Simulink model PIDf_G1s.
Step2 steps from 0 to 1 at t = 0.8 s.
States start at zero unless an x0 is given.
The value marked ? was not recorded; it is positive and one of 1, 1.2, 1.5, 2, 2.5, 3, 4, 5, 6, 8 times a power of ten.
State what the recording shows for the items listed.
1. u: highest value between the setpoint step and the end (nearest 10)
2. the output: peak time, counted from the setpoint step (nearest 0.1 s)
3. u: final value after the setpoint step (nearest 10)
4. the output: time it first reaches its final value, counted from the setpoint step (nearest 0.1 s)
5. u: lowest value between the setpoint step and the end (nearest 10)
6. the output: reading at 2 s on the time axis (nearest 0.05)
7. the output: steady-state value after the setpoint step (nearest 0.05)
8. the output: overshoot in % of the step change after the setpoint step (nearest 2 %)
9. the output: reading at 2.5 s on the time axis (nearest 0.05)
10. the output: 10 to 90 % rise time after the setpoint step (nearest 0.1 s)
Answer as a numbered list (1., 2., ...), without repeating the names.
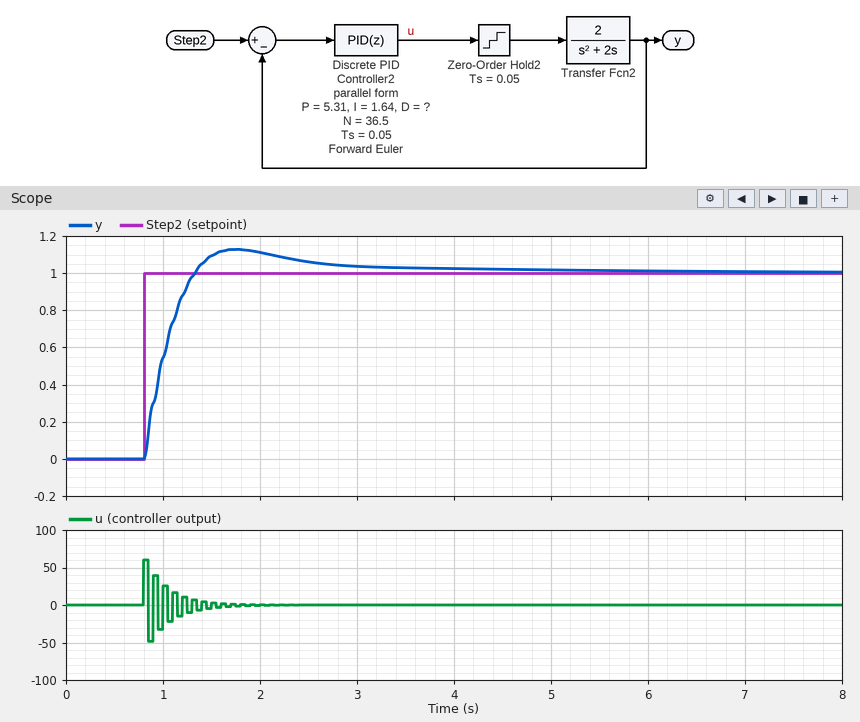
1. 60
2. 1.0 s
3. 0
4. 0.5 s
5. -50
6. 1.10
7. 1.00
8. 12 %
9. 1.05
10. 0.4 s
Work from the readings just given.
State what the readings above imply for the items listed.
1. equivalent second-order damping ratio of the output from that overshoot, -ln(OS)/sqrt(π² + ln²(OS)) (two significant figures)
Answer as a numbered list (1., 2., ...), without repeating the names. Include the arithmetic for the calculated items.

1. ln(0.12) = -2.120; 2.120 / sqrt(9.870 + 4.496) = 0.56
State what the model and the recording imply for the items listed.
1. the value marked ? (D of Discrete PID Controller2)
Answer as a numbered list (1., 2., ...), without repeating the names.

1. 1.5
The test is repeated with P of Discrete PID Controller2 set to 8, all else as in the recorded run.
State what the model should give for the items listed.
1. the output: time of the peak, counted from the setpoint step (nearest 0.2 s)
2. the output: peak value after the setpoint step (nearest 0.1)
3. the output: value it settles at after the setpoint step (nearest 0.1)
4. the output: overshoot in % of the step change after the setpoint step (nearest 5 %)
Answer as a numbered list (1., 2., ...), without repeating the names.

1. 0.6 s
2. 1.2
3. 1.0
4. 20 %
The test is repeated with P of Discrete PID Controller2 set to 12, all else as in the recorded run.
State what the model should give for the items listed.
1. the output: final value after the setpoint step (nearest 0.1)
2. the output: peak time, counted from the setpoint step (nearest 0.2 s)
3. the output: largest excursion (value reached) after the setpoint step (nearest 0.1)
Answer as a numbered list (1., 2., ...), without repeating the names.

1. 1.0
2. 0.6 s
3. 1.3
